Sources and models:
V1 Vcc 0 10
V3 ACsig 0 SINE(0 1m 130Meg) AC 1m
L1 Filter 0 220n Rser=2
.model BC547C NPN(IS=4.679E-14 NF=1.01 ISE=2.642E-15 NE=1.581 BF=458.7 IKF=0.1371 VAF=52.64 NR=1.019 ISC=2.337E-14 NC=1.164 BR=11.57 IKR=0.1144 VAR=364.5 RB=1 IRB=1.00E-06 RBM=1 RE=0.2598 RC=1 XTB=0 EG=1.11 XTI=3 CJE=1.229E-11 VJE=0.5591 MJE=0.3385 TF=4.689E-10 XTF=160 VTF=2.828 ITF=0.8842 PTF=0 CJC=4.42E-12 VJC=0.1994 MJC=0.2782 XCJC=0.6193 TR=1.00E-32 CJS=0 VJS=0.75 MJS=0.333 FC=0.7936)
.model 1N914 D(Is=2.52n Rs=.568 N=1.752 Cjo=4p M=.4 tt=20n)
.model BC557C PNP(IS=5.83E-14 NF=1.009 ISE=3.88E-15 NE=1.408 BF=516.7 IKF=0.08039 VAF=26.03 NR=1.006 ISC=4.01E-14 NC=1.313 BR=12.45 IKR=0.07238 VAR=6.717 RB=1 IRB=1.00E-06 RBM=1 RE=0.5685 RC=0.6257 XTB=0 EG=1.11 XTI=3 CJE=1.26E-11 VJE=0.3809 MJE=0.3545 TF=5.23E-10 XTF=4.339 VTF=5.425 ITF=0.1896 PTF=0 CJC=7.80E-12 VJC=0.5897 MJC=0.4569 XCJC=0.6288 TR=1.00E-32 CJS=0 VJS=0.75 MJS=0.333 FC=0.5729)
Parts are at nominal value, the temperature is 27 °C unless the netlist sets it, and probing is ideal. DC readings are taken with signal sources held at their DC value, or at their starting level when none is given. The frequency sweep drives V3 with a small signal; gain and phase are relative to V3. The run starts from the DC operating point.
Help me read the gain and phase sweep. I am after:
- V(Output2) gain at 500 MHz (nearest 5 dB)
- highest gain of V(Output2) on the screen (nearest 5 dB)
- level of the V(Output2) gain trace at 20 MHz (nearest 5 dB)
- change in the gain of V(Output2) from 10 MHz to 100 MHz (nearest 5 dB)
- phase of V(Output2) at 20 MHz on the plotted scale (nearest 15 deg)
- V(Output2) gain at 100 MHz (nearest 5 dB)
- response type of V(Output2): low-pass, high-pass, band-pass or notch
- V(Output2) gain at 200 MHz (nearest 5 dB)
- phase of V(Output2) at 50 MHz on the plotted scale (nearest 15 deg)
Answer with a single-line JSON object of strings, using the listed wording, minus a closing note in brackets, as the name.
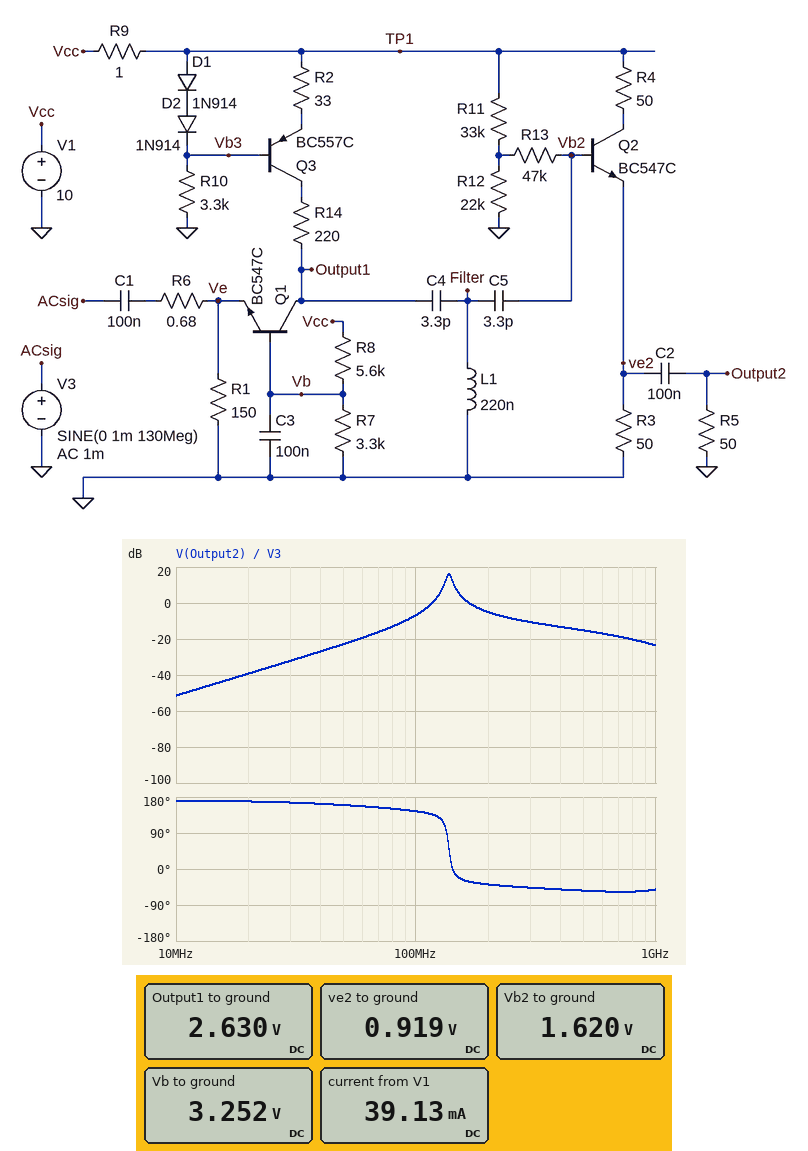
{"V(Output2) gain at 500 MHz": "-15 dB", "highest gain of V(Output2) on the screen": "15 dB", "level of the V(Output2) gain trace at 20 MHz": "-40 dB", "change in the gain of V(Output2) from 10 MHz to 100 MHz": "45 dB", "phase of V(Output2) at 20 MHz on the plotted scale": "165 deg", "V(Output2) gain at 100 MHz": "-5 dB", "response type of V(Output2): low-pass, high-pass, band-pass or notch": "band-pass", "V(Output2) gain at 200 MHz": "-5 dB", "phase of V(Output2) at 50 MHz on the plotted scale": "165 deg"}
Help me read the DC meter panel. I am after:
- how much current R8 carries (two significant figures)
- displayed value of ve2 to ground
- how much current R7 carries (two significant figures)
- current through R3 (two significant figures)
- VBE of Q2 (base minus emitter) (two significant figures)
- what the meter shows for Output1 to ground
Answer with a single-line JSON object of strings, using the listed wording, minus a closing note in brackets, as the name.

{"how much current R8 carries": "1.2 mA", "displayed value of ve2 to ground": "0.919 V", "how much current R7 carries": "990 µA", "current through R3": "18 mA", "VBE of Q2 (base minus emitter)": "700 mV", "what the meter shows for Output1 to ground": "2.630 V"}
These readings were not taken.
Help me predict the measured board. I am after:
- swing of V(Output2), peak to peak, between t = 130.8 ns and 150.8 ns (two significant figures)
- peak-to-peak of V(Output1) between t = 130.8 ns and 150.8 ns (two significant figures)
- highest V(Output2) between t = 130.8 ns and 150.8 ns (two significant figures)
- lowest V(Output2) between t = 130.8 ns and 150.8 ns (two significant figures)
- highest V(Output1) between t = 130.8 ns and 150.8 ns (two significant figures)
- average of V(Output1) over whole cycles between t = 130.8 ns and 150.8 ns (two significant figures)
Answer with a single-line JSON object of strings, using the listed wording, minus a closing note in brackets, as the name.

{"swing of V(Output2), peak to peak, between t = 130.8 ns and 150.8 ns": "5.6 mV", "peak-to-peak of V(Output1) between t = 130.8 ns and 150.8 ns": "9.6 mV", "highest V(Output2) between t = 130.8 ns and 150.8 ns": "2.8 mV", "lowest V(Output2) between t = 130.8 ns and 150.8 ns": "-2.8 mV", "highest V(Output1) between t = 130.8 ns and 150.8 ns": "2.6 V", "average of V(Output1) over whole cycles between t = 130.8 ns and 150.8 ns": "2.6 V"}
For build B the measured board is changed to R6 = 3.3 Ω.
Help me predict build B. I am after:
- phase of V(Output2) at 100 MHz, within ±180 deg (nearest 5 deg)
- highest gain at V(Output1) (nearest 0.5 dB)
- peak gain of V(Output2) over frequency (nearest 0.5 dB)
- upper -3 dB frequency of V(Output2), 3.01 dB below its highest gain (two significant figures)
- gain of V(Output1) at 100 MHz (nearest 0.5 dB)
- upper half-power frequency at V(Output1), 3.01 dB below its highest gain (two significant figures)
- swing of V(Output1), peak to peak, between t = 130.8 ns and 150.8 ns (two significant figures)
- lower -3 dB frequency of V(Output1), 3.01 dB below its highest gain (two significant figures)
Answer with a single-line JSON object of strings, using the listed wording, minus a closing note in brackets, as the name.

{"phase of V(Output2) at 100 MHz, within ±180 deg": "125 deg", "highest gain at V(Output1)": "17.5 dB", "peak gain of V(Output2) over frequency": "11.0 dB", "upper -3 dB frequency of V(Output2), 3.01 dB below its highest gain": "140 MHz", "gain of V(Output1) at 100 MHz": "11.5 dB", "upper half-power frequency at V(Output1), 3.01 dB below its highest gain": "60 MHz", "swing of V(Output1), peak to peak, between t = 130.8 ns and 150.8 ns": "5.0 mV", "lower -3 dB frequency of V(Output1), 3.01 dB below its highest gain": "160 kHz"}
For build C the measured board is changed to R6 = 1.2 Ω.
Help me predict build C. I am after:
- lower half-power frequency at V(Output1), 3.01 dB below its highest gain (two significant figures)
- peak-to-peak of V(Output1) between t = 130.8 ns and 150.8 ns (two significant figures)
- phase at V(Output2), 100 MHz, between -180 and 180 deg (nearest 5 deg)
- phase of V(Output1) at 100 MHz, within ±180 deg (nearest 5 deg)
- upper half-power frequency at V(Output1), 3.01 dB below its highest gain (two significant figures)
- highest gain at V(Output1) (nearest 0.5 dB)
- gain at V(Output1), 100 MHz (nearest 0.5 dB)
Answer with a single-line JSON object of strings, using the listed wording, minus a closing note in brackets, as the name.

{"lower half-power frequency at V(Output1), 3.01 dB below its highest gain": "180 kHz", "peak-to-peak of V(Output1) between t = 130.8 ns and 150.8 ns": "8.2 mV", "phase at V(Output2), 100 MHz, between -180 and 180 deg": "140 deg", "phase of V(Output1) at 100 MHz, within ±180 deg": "-55 deg", "upper half-power frequency at V(Output1), 3.01 dB below its highest gain": "92 MHz", "highest gain at V(Output1)": "18.5 dB", "gain at V(Output1), 100 MHz": "15.0 dB"}
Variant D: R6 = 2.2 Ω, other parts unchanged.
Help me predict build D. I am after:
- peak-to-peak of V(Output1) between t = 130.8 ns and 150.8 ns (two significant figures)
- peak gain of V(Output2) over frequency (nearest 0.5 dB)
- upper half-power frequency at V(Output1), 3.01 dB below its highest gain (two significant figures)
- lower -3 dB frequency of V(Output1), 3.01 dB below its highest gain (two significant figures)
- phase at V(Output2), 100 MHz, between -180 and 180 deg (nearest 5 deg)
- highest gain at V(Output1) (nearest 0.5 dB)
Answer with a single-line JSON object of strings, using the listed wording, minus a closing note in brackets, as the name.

{"peak-to-peak of V(Output1) between t = 130.8 ns and 150.8 ns": "6.3 mV", "peak gain of V(Output2) over frequency": "13.0 dB", "upper half-power frequency at V(Output1), 3.01 dB below its highest gain": "73 MHz", "lower -3 dB frequency of V(Output1), 3.01 dB below its highest gain": "170 kHz", "phase at V(Output2), 100 MHz, between -180 and 180 deg": "130 deg", "highest gain at V(Output1)": "18.0 dB"}
